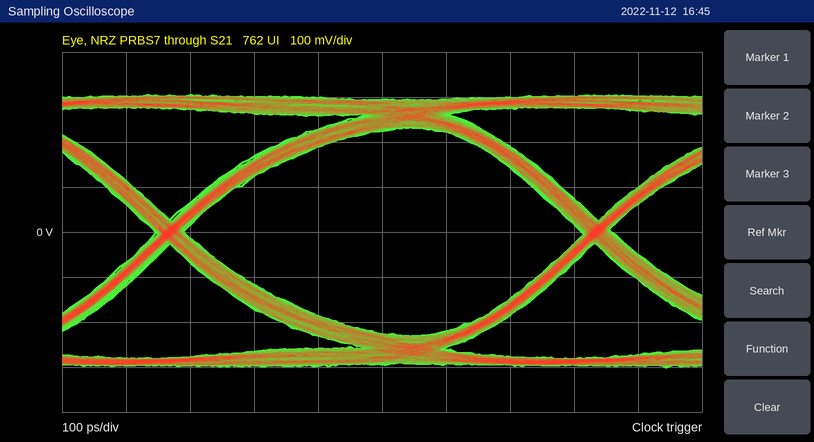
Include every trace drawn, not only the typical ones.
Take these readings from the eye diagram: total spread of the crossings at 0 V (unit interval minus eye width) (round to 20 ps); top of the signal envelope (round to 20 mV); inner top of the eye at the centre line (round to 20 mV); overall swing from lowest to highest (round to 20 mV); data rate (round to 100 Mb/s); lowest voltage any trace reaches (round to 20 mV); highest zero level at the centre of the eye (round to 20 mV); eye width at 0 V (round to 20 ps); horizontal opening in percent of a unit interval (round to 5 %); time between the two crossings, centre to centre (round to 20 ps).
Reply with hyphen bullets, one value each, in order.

- 40 ps
- 300 mV
- 220 mV
- 600 mV
- 1.5 Gb/s
- -300 mV
- -220 mV
- 620 ps
- 95 %
- 660 ps
